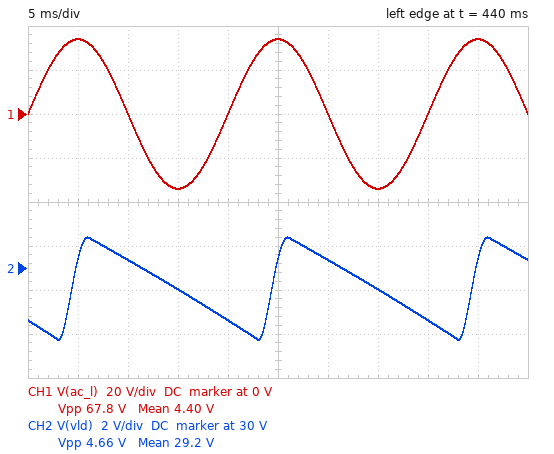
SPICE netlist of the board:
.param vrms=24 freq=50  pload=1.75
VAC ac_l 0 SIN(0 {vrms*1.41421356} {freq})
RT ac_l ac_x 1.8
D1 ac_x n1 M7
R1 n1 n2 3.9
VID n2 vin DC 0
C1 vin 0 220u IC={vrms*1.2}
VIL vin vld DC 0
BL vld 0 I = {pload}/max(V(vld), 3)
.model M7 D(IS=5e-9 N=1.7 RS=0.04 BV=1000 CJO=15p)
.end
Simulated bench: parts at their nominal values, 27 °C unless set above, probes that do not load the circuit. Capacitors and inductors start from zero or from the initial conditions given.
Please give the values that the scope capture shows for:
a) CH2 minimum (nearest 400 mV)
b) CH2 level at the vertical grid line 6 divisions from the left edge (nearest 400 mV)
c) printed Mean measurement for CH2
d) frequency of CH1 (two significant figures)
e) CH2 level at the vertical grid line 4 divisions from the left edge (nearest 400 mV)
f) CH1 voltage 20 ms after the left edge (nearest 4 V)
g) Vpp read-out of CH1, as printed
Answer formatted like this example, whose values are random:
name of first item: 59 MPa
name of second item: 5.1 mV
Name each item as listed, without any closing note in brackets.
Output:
CH2 minimum: 26.8 V
CH2 level at the vertical grid line 6 divisions from the left edge: 30.4 V
printed Mean measurement for CH2: 29.2 V
frequency of CH1: 50 Hz
CH2 level at the vertical grid line 4 divisions from the left edge: 27.6 V
CH1 voltage 20 ms after the left edge: 0 V
Vpp read-out of CH1, as printed: 67.8 V
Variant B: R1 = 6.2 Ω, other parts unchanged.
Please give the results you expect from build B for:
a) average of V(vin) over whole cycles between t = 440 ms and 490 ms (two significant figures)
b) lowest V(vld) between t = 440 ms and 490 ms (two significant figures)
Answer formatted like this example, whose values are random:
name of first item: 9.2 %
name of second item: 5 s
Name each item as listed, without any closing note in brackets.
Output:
average of V(vin) over whole cycles between t = 440 ms and 490 ms: 28 V
lowest V(vld) between t = 440 ms and 490 ms: 26 V
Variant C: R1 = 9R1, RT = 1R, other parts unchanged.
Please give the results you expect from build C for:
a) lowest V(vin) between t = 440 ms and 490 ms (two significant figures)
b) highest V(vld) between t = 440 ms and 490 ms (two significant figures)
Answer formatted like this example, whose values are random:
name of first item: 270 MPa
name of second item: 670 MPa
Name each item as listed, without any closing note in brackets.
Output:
lowest V(vin) between t = 440 ms and 490 ms: 25 V
highest V(vld) between t = 440 ms and 490 ms: 30 V
